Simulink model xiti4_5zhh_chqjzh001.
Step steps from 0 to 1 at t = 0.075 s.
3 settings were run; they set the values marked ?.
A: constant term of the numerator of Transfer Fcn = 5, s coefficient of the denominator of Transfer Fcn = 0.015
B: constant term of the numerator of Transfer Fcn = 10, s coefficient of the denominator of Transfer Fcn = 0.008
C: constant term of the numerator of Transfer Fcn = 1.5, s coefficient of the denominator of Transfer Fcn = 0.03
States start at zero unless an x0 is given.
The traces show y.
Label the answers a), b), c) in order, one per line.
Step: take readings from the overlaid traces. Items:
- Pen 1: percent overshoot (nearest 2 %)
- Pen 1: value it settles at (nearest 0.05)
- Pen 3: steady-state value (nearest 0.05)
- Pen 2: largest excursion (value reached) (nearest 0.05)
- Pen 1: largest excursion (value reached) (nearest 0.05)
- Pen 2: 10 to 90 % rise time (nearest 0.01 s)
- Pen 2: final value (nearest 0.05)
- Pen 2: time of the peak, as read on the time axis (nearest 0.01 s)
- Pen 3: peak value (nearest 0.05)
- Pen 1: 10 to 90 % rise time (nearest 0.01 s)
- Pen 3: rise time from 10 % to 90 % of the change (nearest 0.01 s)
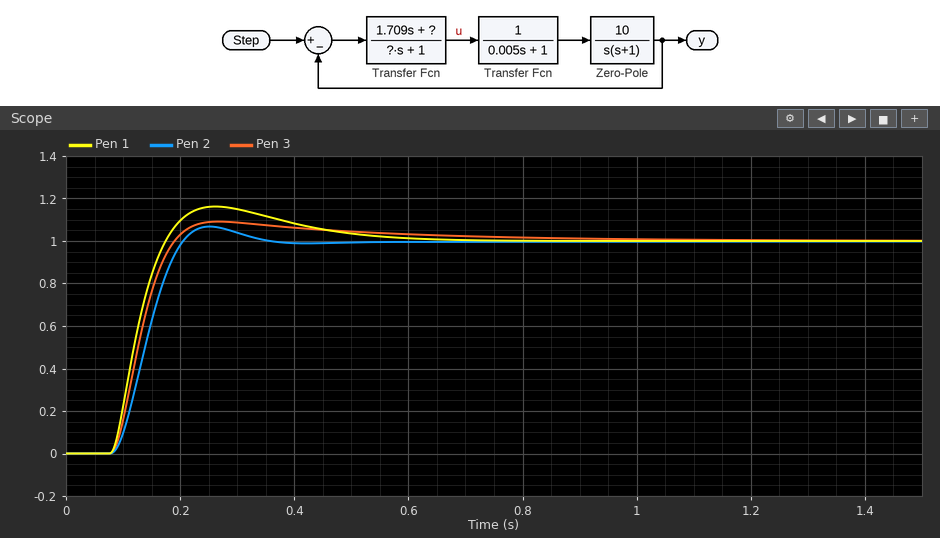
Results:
a) 16 %
b) 1.00
c) 1.00
d) 1.05
e) 1.15
f) 0.08 s
g) 1.00
h) 0.25 s
i) 1.10
j) 0.07 s
k) 0.07 s
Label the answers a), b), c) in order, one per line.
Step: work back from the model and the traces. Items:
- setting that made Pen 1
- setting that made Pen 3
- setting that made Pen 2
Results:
a) B
b) A
c) C
